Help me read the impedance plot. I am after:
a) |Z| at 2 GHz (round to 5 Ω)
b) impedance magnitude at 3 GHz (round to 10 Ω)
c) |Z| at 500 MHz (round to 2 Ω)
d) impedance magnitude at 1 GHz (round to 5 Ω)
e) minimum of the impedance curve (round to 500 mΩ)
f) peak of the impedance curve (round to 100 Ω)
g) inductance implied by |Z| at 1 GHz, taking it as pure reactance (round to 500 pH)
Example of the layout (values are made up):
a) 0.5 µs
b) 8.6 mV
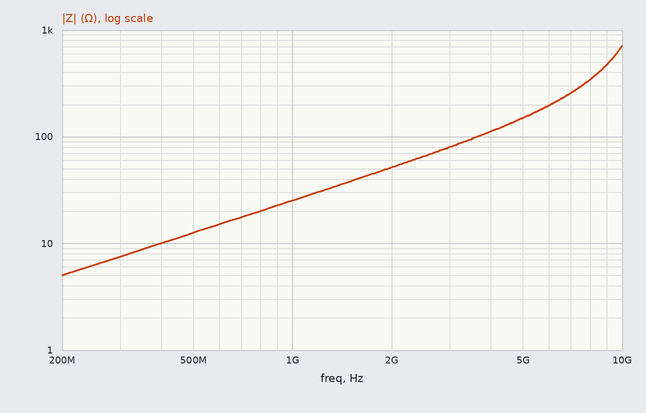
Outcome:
a) 50 Ω
b) 80 Ω
c) 12 Ω
d) 25 Ω
e) 5.0 Ω
f) 700 Ω
g) 4.0 nH
